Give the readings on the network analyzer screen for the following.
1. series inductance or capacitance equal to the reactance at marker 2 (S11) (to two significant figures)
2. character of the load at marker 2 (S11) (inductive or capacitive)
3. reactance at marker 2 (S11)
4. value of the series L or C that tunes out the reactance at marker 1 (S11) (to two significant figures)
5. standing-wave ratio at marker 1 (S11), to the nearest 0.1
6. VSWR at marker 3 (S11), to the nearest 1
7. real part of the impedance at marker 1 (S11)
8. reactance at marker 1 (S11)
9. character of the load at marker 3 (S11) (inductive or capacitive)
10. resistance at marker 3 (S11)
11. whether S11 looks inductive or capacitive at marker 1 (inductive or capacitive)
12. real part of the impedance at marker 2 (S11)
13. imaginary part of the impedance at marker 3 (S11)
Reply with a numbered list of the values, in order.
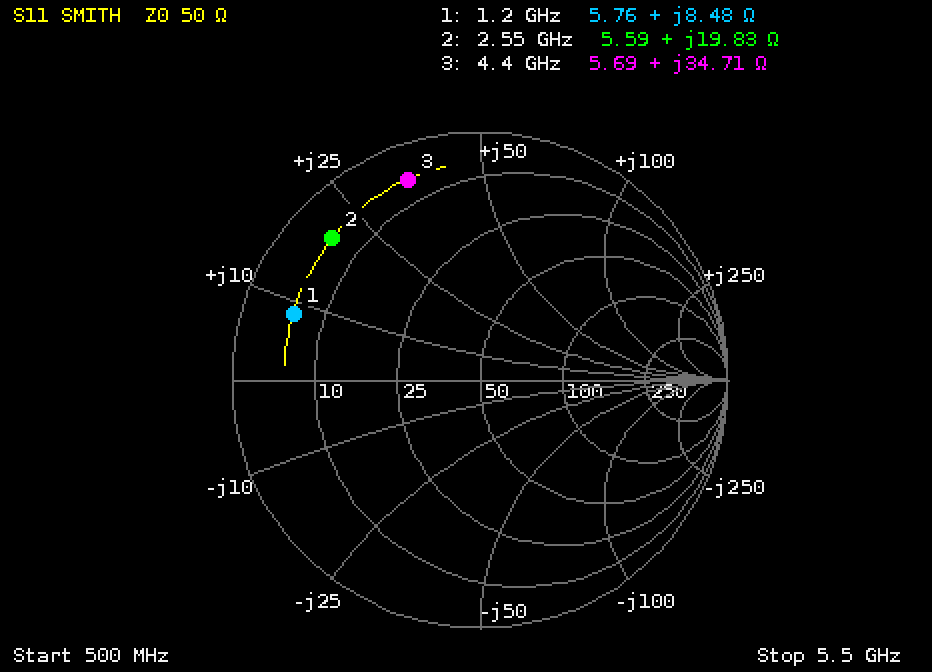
1. 1.2 nH
2. inductive
3. +19.83 Ω
4. 16 pF
5. 8.9
6. 13
7. 5.76 Ω
8. +8.48 Ω
9. inductive
10. 5.69 Ω
11. inductive
12. 5.59 Ω
13. +34.71 Ω
